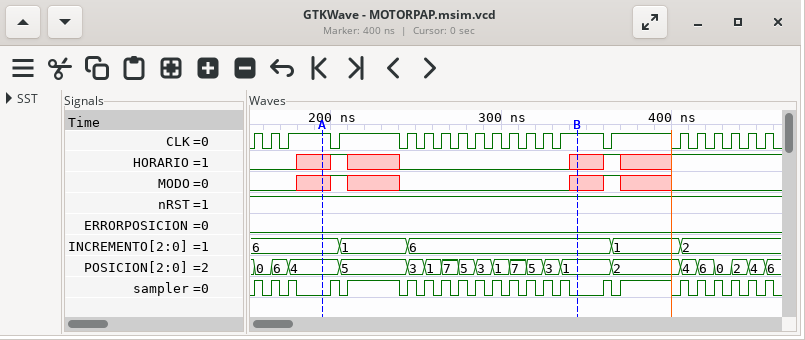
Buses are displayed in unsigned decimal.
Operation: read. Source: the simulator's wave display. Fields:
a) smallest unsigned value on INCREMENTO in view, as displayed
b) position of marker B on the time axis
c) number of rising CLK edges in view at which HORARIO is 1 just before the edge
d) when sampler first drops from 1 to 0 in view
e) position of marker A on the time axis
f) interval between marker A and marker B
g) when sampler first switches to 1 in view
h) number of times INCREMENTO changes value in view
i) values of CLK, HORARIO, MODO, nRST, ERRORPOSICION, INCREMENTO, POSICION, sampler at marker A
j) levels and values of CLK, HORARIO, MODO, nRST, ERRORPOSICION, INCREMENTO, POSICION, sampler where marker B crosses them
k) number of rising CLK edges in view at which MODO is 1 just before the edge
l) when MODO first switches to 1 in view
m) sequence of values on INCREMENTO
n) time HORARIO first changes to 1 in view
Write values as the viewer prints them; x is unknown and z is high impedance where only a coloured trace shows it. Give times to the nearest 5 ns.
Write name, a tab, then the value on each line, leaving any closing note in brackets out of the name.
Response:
smallest unsigned value on INCREMENTO in view, as displayed	1
position of marker B on the time axis	345 ns
number of rising CLK edges in view at which HORARIO is 1 just before the edge	8
when sampler first drops from 1 to 0 in view	160 ns
position of marker A on the time axis	195 ns
interval between marker A and marker B	150 ns
when sampler first switches to 1 in view	155 ns
number of times INCREMENTO changes value in view	4
values of CLK, HORARIO, MODO, nRST, ERRORPOSICION, INCREMENTO, POSICION, sampler at marker A	CLK=1, HORARIO=x, MODO=x, nRST=1, ERRORPOSICION=0, INCREMENTO=6, POSICION=4, sampler=0
levels and values of CLK, HORARIO, MODO, nRST, ERRORPOSICION, INCREMENTO, POSICION, sampler where marker B crosses them	CLK=1, HORARIO=x, MODO=x, nRST=1, ERRORPOSICION=0, INCREMENTO=6, POSICION=1, sampler=0
number of rising CLK edges in view at which MODO is 1 just before the edge	2
when MODO first switches to 1 in view	200 ns
sequence of values on INCREMENTO	6, 1, 6, 1, 2
time HORARIO first changes to 1 in view	200 ns
